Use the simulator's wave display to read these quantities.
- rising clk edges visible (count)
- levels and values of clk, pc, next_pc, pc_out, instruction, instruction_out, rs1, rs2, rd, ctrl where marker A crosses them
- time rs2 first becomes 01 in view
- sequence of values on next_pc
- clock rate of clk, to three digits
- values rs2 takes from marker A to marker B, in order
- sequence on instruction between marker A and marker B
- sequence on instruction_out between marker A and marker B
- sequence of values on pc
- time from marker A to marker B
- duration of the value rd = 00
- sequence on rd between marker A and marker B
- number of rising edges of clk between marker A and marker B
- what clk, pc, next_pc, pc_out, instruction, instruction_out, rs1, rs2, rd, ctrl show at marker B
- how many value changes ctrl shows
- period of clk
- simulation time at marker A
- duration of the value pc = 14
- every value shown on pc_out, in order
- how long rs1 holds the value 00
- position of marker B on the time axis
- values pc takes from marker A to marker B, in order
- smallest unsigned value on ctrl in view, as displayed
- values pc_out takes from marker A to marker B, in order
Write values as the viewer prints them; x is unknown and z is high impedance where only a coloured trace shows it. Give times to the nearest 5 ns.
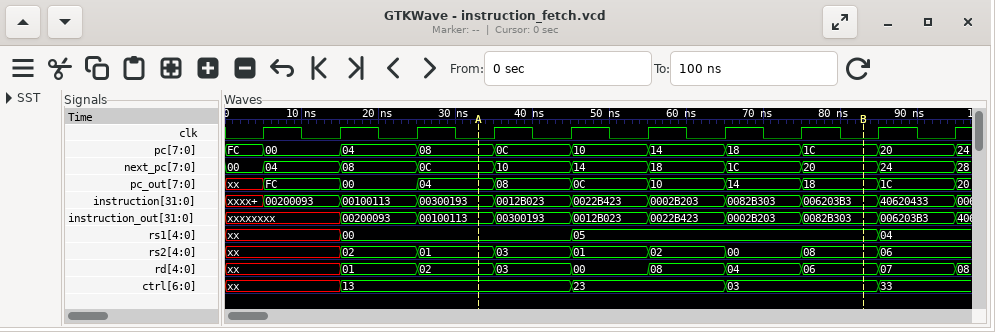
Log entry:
10
clk=0, pc=08, next_pc=0C, pc_out=04, instruction=00300193, instruction_out=00100113, rs1=00, rs2=01, rd=02, ctrl=13
25 ns
00, 04, 08, 0C, 10, 14, 18, 1C, 20, 24, 28
100 MHz
01, 03, 01, 02, 00, 08
00300193, 0012B023, 0022B423, 0002B203, 0082B303, 006203B3
00100113, 00300193, 0012B023, 0022B423, 0002B203, 0082B303
FC, 00, 04, 08, 0C, 10, 14, 18, 1C, 20, 24
50 ns
10 ns
02, 03, 00, 08, 04, 06
5
clk=0, pc=1C, next_pc=20, pc_out=18, instruction=006203B3, instruction_out=0082B303, rs1=05, rs2=08, rd=06, ctrl=03
4
10 ns
35 ns
10 ns
xx, FC, 00, 04, 08, 0C, 10, 14, 18, 1C, 20
30 ns
85 ns
08, 0C, 10, 14, 18, 1C
03
04, 08, 0C, 10, 14, 18
